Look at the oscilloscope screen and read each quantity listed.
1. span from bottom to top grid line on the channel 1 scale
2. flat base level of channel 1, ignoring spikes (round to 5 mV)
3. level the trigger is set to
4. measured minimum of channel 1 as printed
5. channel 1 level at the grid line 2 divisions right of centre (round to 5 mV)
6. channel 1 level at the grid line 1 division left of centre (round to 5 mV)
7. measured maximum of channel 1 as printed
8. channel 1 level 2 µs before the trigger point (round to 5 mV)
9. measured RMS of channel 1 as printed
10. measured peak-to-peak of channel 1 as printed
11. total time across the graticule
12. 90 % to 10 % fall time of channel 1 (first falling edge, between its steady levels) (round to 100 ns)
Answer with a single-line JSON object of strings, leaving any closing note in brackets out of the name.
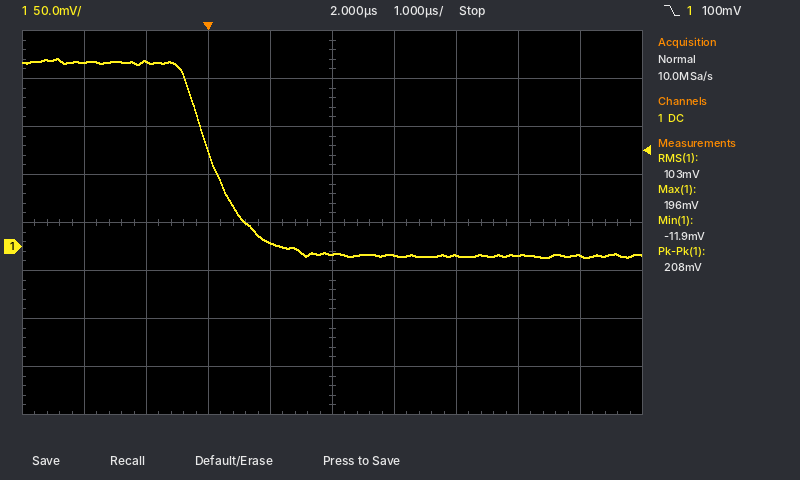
{"span from bottom to top grid line on the channel 1 scale": "400 mV", "flat base level of channel 1, ignoring spikes": "-10 mV", "level the trigger is set to": "100 mV", "measured minimum of channel 1 as printed": "-11.9 mV", "channel 1 level at the grid line 2 divisions right of centre": "-10 mV", "channel 1 level at the grid line 1 division left of centre": "5 mV", "measured maximum of channel 1 as printed": "196 mV", "channel 1 level 2 µs before the trigger point": "190 mV", "measured RMS of channel 1 as printed": "103 mV", "measured peak-to-peak of channel 1 as printed": "208 mV", "total time across the graticule": "10 µs", "90 % to 10 % fall time of channel 1 (first falling edge, between its steady levels)": "1.2 µs"}
